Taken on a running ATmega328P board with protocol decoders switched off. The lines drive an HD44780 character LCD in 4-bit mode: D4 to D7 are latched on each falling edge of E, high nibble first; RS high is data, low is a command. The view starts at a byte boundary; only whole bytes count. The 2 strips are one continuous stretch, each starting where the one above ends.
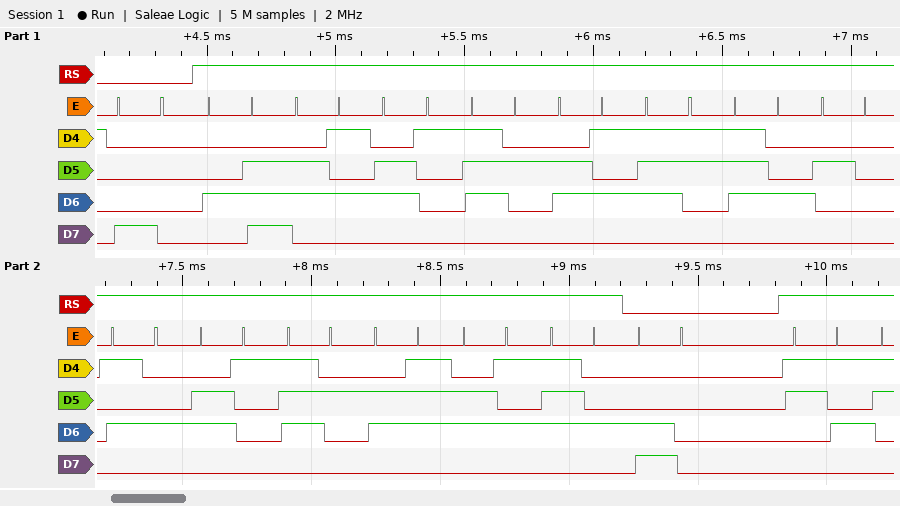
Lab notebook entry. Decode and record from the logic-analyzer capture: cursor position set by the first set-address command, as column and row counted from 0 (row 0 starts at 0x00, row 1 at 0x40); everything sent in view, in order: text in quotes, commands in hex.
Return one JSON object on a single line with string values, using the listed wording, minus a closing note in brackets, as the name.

{"cursor position set by the first set-address command, as column and row counted from 0": "column 0, row 0", "everything sent in view, in order: text in quotes, commands in hex": "0x80 \"Nearest Target\" 0xC0 \"5\""}
